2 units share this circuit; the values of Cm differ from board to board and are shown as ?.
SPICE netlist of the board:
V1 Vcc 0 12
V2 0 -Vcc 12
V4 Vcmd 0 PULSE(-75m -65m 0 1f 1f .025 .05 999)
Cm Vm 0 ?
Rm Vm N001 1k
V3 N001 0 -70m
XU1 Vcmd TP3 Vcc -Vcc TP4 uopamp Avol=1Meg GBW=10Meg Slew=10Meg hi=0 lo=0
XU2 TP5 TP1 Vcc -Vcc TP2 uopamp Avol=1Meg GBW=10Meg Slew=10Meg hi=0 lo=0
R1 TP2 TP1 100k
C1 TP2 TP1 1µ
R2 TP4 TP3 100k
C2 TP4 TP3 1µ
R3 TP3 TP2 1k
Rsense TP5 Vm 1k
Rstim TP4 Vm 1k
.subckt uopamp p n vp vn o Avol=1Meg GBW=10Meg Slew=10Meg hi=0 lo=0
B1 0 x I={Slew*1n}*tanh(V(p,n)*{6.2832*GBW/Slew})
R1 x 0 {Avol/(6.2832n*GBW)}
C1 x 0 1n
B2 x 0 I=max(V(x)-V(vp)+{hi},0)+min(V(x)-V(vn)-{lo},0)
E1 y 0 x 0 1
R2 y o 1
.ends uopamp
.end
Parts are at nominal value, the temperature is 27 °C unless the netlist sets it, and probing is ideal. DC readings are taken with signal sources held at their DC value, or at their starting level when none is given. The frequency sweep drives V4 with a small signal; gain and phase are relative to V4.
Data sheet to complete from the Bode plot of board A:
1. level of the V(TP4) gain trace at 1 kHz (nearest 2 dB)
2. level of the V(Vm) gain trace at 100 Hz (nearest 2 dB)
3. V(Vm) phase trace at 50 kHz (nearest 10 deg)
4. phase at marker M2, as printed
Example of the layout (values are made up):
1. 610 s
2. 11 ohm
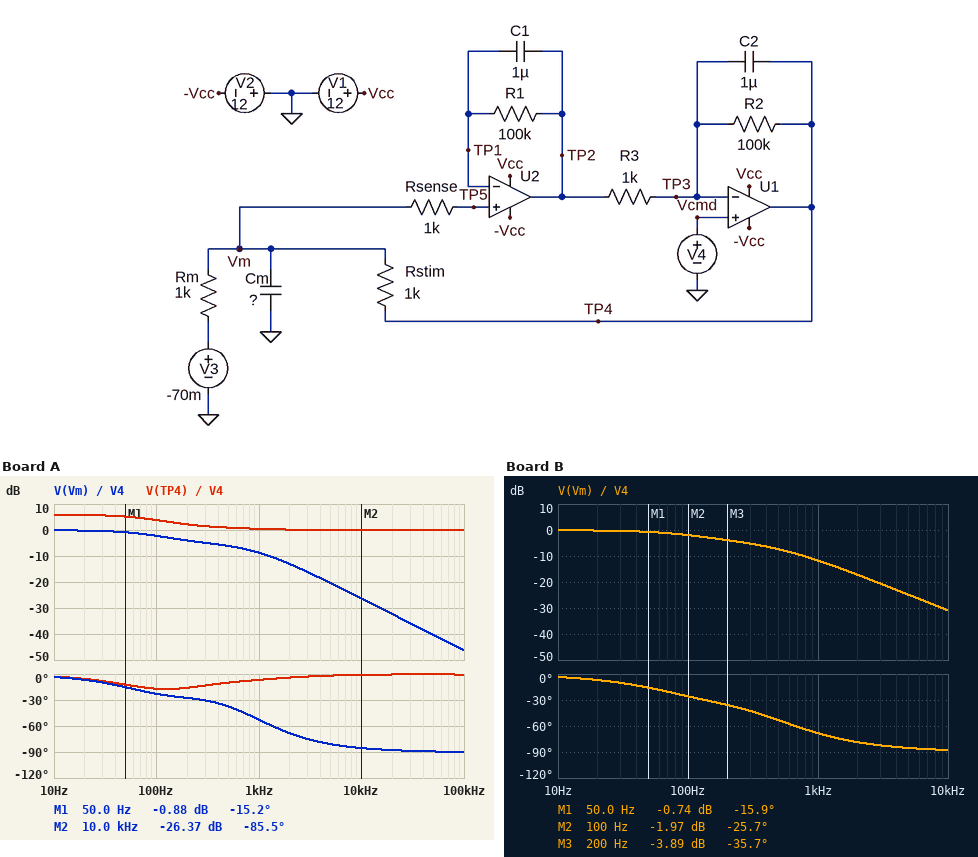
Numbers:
1. 0 dB
2. -2 dB
3. -90 deg
4. -85.5 deg
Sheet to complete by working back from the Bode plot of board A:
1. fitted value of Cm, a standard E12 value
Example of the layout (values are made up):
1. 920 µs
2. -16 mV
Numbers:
1. 330 nF
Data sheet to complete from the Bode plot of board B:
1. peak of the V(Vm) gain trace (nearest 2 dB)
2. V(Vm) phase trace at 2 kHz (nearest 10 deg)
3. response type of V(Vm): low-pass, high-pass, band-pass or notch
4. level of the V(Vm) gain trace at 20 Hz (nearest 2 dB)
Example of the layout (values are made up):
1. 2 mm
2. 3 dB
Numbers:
1. 0 dB
2. -80 deg
3. low-pass
4. 0 dB
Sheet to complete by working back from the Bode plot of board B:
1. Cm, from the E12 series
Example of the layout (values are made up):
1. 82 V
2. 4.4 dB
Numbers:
1. 560 nF
